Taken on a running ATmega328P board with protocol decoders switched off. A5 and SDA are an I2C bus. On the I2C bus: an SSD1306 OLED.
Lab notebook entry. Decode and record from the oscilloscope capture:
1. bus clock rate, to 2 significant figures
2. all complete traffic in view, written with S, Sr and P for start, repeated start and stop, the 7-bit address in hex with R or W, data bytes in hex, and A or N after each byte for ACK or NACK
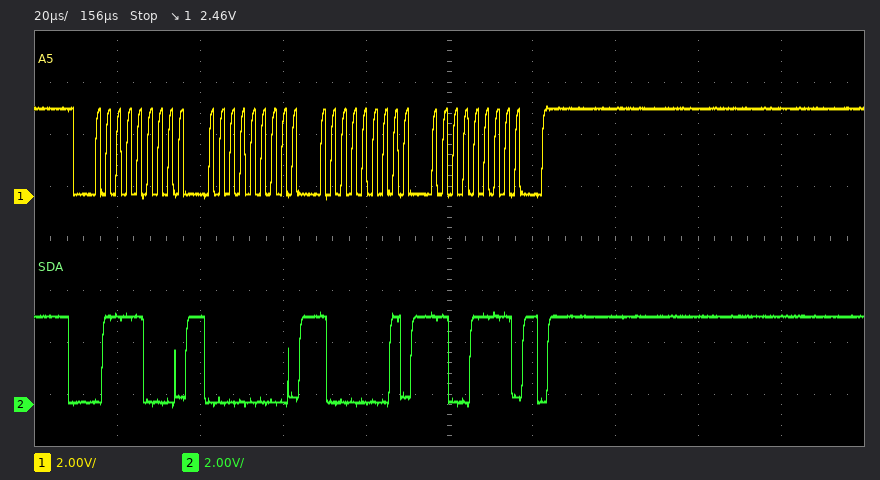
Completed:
400 kHz
S 3CW A 00 A 81 A CF A P
